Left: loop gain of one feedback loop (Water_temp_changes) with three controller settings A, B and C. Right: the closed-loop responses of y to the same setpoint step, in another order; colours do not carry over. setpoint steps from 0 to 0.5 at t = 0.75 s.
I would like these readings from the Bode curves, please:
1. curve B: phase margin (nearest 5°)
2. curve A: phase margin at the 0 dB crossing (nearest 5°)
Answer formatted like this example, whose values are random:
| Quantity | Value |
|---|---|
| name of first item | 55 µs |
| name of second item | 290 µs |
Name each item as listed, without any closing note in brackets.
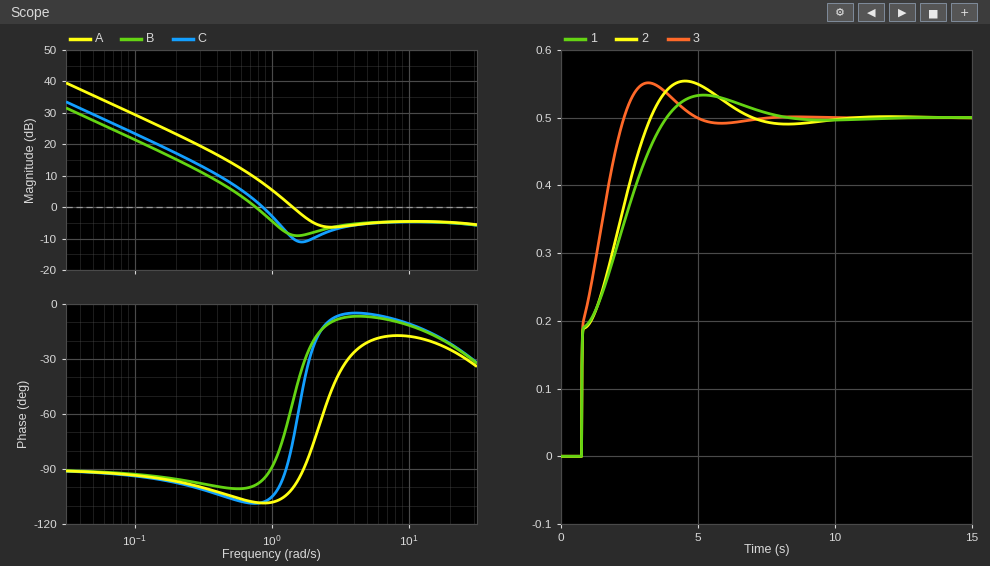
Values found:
| Quantity | Value |
|---|---|
| curve B: phase margin | 80° |
| curve A: phase margin at the 0 dB crossing | 80° |
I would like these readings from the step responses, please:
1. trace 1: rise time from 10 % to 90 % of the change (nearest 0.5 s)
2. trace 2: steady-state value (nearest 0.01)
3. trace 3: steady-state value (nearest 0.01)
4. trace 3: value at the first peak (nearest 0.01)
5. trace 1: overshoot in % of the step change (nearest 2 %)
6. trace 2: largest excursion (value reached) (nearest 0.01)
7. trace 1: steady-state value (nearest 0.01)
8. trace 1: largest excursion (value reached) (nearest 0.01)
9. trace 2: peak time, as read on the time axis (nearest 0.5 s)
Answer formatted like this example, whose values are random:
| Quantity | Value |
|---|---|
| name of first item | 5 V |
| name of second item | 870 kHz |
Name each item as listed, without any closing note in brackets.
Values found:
| Quantity | Value |
|---|---|
| trace 1: rise time from 10 % to 90 % of the change | 2.5 s |
| trace 2: steady-state value | 0.50 |
| trace 3: steady-state value | 0.50 |
| trace 3: value at the first peak | 0.55 |
| trace 1: overshoot in % of the step change | 6 % |
| trace 2: largest excursion (value reached) | 0.55 |
| trace 1: steady-state value | 0.50 |
| trace 1: largest excursion (value reached) | 0.53 |
| trace 2: peak time, as read on the time axis | 4.5 s |
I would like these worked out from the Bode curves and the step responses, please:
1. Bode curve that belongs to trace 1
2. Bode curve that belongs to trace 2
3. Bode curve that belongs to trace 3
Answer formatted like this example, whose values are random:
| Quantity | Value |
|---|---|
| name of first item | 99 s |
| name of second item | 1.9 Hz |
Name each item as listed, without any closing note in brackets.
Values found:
| Quantity | Value |
|---|---|
| Bode curve that belongs to trace 1 | B |
| Bode curve that belongs to trace 2 | C |
| Bode curve that belongs to trace 3 | A |
